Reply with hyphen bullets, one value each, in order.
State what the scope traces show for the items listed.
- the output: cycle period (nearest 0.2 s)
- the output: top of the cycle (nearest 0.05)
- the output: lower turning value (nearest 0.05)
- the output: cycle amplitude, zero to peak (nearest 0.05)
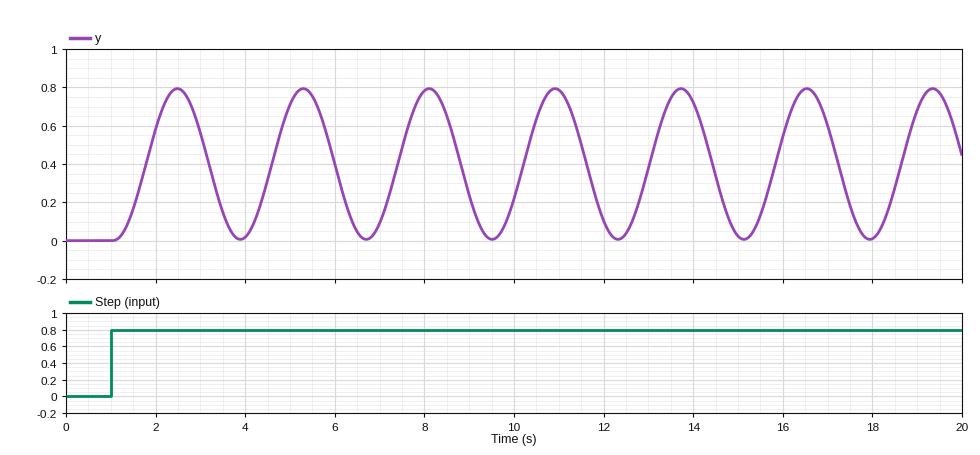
- 2.8 s
- 0.80
- 0.00
- 0.40
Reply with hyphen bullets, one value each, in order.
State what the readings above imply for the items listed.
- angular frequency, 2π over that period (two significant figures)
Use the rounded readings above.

- 2.2 rad/s
